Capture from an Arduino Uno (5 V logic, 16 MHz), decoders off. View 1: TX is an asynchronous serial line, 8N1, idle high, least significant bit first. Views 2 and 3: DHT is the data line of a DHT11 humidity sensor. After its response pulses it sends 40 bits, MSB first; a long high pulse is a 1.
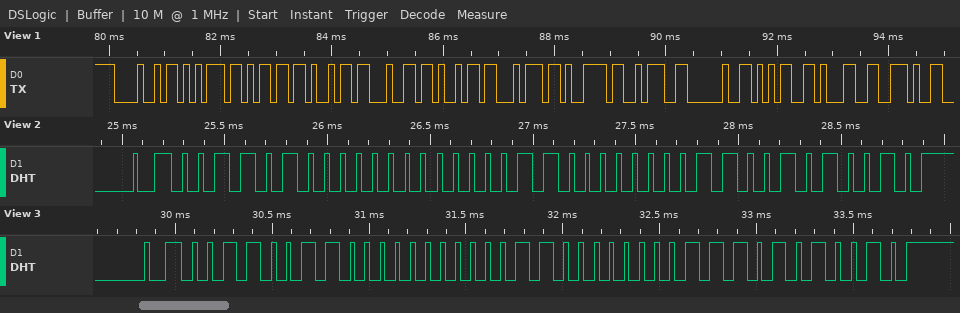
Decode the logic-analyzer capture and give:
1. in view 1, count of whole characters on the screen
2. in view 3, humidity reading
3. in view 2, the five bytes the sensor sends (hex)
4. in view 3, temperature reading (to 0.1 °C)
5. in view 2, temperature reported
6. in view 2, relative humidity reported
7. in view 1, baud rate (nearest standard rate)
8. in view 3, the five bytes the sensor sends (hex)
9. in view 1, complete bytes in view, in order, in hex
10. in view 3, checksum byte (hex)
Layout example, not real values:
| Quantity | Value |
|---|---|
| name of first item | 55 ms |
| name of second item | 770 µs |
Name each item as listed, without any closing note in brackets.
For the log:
| Quantity | Value |
|---|---|
| in view 1, count of whole characters on the screen | 13 |
| in view 3, humidity reading | 51 % |
| in view 2, the five bytes the sensor sends | 34 00 18 06 52 |
| in view 3, temperature reading | 24.7 °C |
| in view 2, temperature reported | 24.6 °C |
| in view 2, relative humidity reported | 52 % |
| in view 1, baud rate | 9600 baud |
| in view 3, the five bytes the sensor sends | 33 00 18 07 52 |
| in view 1, complete bytes in view, in order, in hex | 48 75 6D 69 64 69 74 79 3A 20 35 31 2E |
| in view 3, checksum byte | 0x52 |
